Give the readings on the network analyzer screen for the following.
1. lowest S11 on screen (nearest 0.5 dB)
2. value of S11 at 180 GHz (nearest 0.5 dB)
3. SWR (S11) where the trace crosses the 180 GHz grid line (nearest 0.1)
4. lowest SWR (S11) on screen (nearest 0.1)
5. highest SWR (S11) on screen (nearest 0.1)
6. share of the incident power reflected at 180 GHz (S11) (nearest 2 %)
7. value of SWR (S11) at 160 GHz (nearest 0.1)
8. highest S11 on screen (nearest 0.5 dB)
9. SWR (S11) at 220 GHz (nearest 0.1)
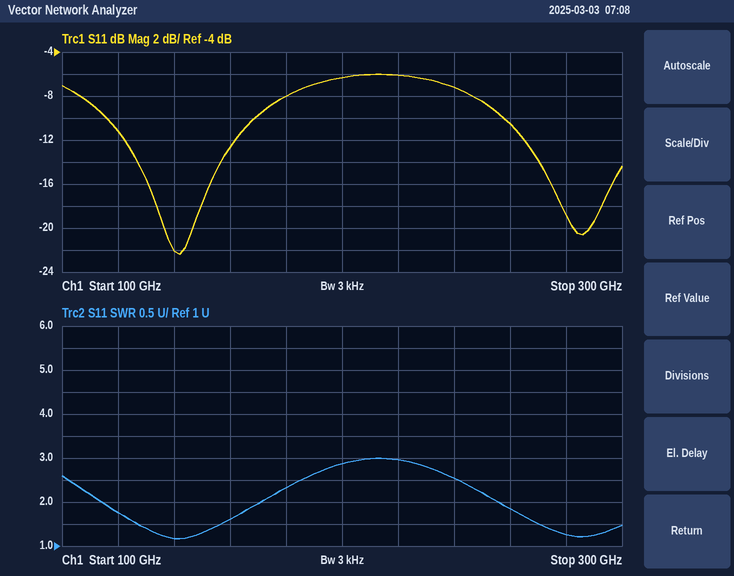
-22.5 dB
-8.0 dB
2.3
1.2
3.0
16 %
1.6
-6.0 dB
3.0
